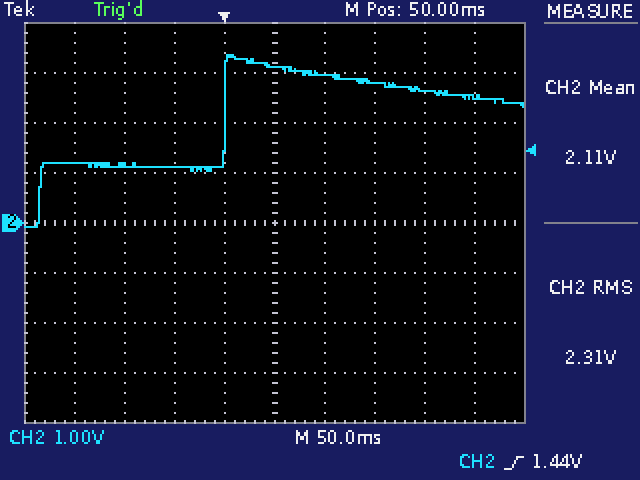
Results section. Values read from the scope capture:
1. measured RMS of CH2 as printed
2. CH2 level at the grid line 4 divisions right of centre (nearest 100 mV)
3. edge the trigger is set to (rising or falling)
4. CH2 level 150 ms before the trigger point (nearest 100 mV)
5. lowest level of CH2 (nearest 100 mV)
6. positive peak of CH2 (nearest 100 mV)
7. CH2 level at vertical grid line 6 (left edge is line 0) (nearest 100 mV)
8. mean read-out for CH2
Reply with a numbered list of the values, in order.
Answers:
1. 2.31 V
2. 2.5 V
3. rising
4. 1.2 V
5. -100 mV
6. 3.4 V
7. 3.0 V
8. 2.11 V
